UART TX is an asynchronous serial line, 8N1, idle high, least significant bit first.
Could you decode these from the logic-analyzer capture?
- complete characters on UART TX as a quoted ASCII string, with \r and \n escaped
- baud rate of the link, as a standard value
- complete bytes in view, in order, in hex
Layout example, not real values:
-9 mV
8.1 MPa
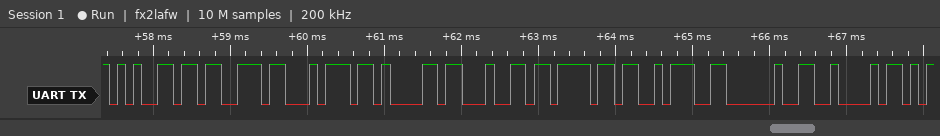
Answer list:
"estado: B"
9600 baud
0x65 0x73 0x74 0x61 0x64 0x6F 0x3A 0x20 0x42
